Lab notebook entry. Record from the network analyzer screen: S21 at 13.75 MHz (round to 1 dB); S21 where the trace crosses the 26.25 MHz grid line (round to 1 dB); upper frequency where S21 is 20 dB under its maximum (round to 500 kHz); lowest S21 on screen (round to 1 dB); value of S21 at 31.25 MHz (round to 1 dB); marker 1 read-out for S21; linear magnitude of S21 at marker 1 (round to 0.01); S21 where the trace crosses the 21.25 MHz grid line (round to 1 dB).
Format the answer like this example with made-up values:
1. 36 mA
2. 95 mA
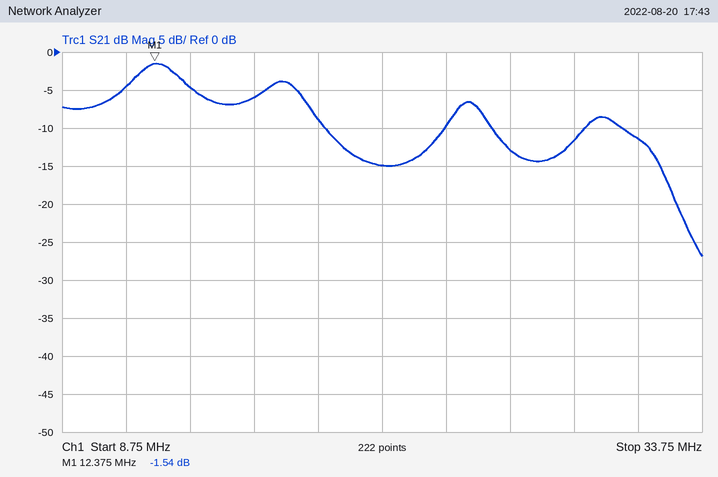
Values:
1. -5 dB
2. -13 dB
3. 33.0 MHz
4. -27 dB
5. -11 dB
6. -1.54 dB
7. 0.84
8. -15 dB
